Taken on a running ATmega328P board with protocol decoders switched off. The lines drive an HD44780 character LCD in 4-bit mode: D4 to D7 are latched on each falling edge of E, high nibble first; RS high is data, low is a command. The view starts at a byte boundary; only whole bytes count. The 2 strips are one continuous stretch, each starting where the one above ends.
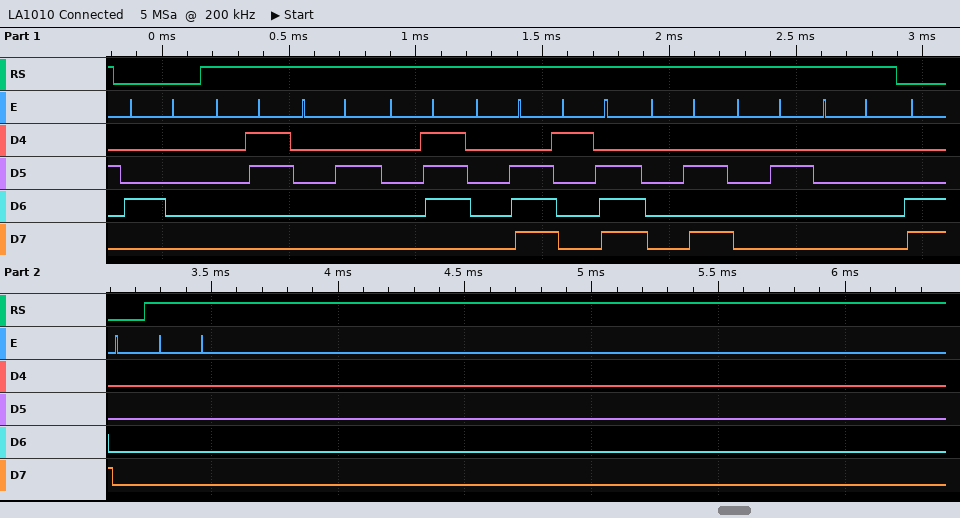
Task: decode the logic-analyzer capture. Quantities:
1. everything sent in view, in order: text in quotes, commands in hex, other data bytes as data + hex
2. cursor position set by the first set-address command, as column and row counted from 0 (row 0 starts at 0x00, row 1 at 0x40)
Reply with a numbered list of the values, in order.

1. 0x40 data 03 02 07 0E 1E 0A 02 00 0xC0 data 00
2. column 0, row 1
